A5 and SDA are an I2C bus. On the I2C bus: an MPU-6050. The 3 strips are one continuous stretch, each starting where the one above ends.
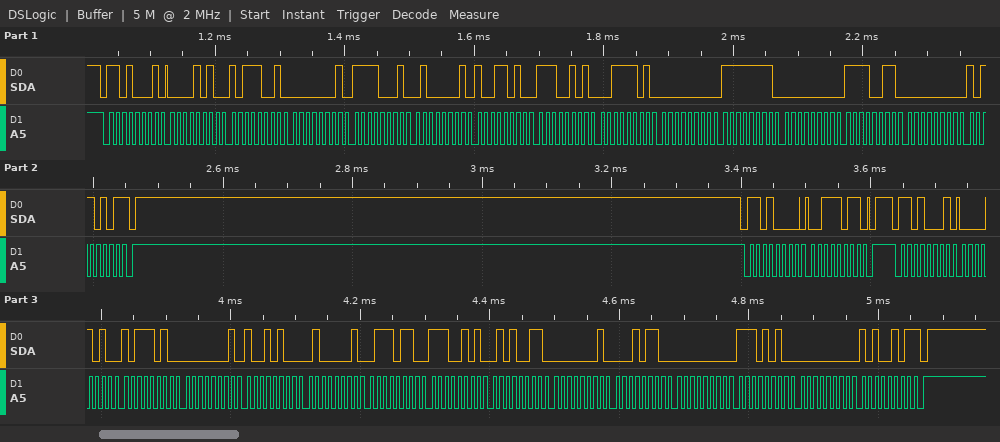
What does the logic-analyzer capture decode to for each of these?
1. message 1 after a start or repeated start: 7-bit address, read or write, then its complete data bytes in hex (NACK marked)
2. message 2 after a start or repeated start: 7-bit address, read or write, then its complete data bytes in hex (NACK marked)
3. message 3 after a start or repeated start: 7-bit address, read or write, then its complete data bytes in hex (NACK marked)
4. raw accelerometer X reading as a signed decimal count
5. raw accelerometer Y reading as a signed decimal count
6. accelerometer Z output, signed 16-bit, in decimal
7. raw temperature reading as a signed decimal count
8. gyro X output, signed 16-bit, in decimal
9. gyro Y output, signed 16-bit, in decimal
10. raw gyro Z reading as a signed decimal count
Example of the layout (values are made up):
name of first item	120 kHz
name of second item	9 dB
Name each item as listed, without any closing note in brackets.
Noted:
message 1 after a start or repeated start: 7-bit address, read or write, then its complete data bytes in hex	0x68 read: 0A B9 01 F1 41 9A E5 3D 00 FF 00 F3 00 B5 NACK
message 2 after a start or repeated start: 7-bit address, read or write, then its complete data bytes in hex	0x68 write: 3B
message 3 after a start or repeated start: 7-bit address, read or write, then its complete data bytes in hex	0x68 read: 0A BA 01 94 41 76 E5 53 01 16 00 EA 00 A5 NACK
raw accelerometer X reading as a signed decimal count	2746
raw accelerometer Y reading as a signed decimal count	404
accelerometer Z output, signed 16-bit, in decimal	16758
raw temperature reading as a signed decimal count	-6829
gyro X output, signed 16-bit, in decimal	278
gyro Y output, signed 16-bit, in decimal	234
raw gyro Z reading as a signed decimal count	165
